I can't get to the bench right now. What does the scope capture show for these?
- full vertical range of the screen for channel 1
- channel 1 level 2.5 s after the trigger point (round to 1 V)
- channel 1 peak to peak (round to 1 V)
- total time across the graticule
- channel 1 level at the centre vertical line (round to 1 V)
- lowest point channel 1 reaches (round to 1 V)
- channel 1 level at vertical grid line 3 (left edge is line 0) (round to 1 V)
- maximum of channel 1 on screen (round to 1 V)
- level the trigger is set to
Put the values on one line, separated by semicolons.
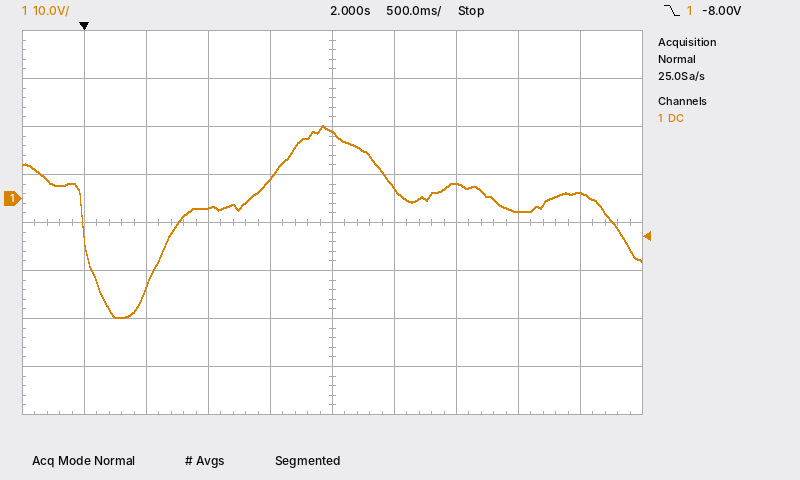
80 V; 2 V; 40 V; 5 s; 14 V; -25 V; -2 V; 15 V; -8.00 V
